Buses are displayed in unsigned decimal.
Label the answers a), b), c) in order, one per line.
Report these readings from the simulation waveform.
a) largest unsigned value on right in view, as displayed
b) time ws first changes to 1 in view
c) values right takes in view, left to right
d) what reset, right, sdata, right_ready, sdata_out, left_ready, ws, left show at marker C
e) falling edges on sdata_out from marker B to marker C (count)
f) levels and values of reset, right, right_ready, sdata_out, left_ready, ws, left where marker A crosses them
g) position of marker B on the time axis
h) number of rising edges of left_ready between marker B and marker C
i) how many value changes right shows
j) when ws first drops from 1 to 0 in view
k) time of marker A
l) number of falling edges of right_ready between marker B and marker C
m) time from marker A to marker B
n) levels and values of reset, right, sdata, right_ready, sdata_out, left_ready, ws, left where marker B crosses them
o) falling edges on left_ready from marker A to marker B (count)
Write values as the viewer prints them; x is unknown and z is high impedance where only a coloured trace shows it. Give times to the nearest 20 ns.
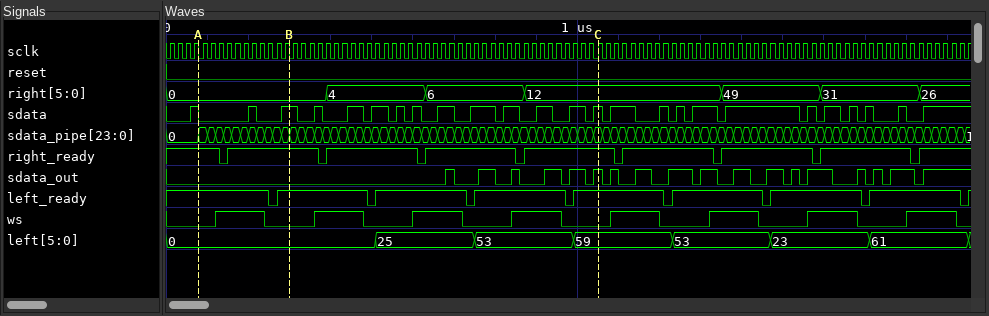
a) 49
b) 120 ns
c) 0, 4, 6, 12, 49, 31, 26
d) reset=0, right=12, sdata=1, right_ready=1, sdata_out=1, left_ready=1, ws=0, left=59
e) 5
f) reset=0, right=0, right_ready=1, sdata_out=0, left_ready=1, ws=0, left=0
g) 300 ns
h) 3
i) 6
j) 240 ns
k) 80 ns
l) 3
m) 220 ns
n) reset=0, right=0, sdata=1, right_ready=1, sdata_out=0, left_ready=1, ws=0, left=0
o) 1
